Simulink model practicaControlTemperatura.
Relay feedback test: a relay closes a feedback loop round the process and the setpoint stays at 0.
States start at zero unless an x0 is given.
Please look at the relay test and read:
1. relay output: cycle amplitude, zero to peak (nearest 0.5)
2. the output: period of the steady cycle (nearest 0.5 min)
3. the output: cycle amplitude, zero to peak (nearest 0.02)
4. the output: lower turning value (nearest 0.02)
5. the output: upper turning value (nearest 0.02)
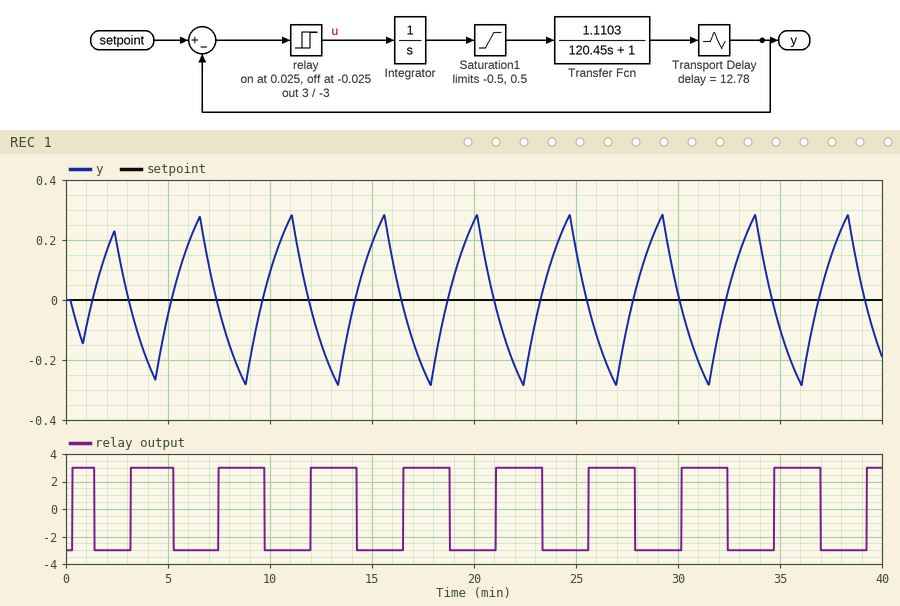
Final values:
3.0
4.5 min
0.28
-0.28
0.28
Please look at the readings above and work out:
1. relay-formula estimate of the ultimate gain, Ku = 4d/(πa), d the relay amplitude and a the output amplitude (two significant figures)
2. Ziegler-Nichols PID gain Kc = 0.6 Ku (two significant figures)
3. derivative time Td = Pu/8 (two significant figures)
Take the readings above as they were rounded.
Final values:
14
8.4
0.56 min
